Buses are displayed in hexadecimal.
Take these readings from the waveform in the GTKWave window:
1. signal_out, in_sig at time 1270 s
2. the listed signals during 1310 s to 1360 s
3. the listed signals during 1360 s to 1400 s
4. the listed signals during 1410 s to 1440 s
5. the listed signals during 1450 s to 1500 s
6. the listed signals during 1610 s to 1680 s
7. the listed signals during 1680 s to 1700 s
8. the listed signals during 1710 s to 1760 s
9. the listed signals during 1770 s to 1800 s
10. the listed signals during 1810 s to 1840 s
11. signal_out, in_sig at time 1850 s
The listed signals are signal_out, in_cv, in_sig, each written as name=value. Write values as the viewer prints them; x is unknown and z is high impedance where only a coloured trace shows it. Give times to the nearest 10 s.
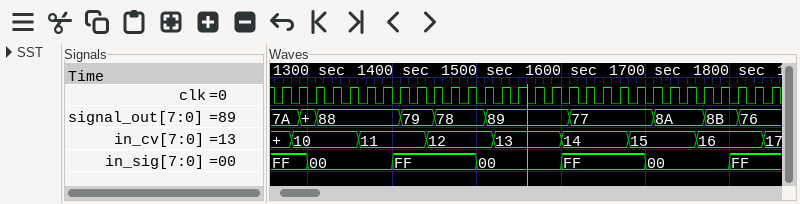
signal_out=7A, in_sig=FF
signal_out=88, in_cv=10, in_sig=00
signal_out=88, in_cv=11, in_sig=00
signal_out=79, in_cv=11, in_sig=FF
signal_out=78, in_cv=12, in_sig=FF
signal_out=77, in_cv=14, in_sig=FF
signal_out=77, in_cv=15, in_sig=FF
signal_out=8A, in_cv=15, in_sig=00
signal_out=8B, in_cv=16, in_sig=00
signal_out=76, in_cv=16, in_sig=FF
signal_out=76, in_sig=FF
